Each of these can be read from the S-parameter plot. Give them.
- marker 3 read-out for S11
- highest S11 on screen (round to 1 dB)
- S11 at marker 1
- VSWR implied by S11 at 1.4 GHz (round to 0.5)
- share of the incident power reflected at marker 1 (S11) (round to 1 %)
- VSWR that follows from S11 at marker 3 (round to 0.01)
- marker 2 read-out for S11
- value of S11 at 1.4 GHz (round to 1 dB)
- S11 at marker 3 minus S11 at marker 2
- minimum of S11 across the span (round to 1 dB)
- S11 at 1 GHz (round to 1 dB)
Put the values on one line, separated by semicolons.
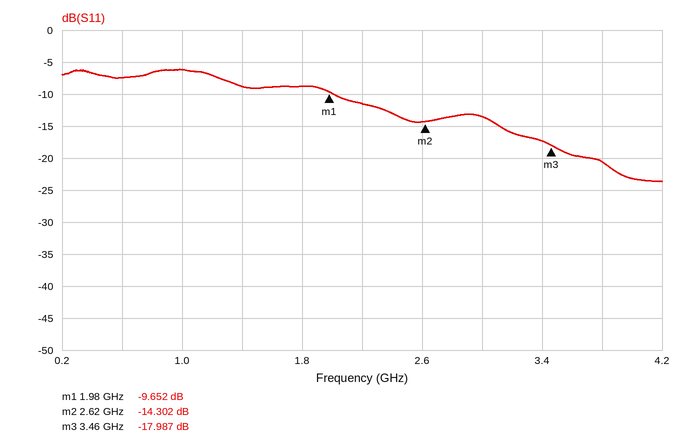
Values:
-17.987 dB; -6 dB; -9.652 dB; 2.0; 11 %; 1.29; -14.302 dB; -9 dB; -3.685 dB; -24 dB; -6 dB
